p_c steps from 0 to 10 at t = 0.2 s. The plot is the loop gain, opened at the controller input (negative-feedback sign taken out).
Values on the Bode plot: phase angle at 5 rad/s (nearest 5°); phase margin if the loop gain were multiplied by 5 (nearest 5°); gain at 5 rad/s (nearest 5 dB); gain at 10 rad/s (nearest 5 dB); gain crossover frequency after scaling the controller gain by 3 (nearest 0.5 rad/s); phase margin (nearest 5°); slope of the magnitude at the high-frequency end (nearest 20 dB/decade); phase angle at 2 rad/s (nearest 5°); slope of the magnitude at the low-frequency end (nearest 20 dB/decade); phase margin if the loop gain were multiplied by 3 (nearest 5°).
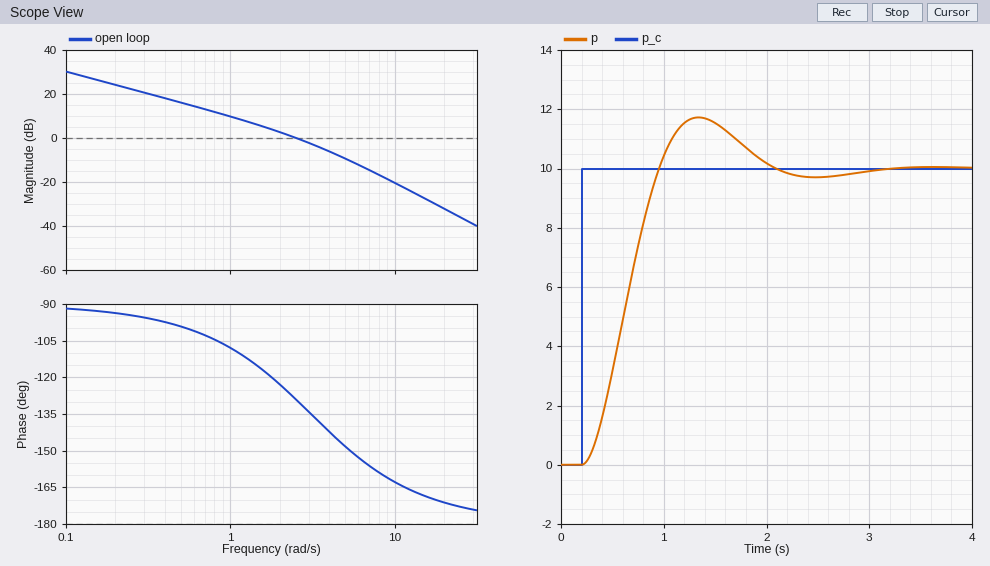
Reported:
-150°
25°
-10 dB
-20 dB
5.0 rad/s
50°
-40 dB/decade
-125°
-20 dB/decade
30°
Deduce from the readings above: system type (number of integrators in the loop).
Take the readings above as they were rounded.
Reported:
1
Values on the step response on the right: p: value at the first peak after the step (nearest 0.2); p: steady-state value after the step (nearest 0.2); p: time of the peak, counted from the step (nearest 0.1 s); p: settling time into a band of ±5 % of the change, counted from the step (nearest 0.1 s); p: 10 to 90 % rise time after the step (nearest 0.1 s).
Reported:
11.8
10.0
1.1 s
1.7 s
0.5 s
